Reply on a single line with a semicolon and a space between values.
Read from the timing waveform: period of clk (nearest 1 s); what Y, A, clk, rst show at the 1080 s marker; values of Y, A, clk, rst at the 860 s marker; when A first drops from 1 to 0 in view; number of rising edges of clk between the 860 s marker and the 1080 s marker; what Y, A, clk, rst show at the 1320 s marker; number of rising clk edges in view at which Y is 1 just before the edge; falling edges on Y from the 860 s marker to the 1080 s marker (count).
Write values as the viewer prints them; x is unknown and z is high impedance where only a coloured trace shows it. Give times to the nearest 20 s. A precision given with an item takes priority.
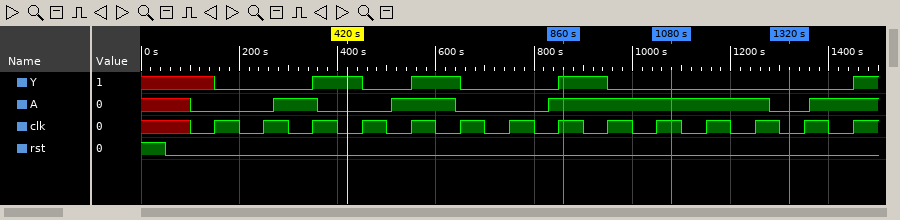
100 s; Y=0, A=1, clk=1, rst=0; Y=1, A=1, clk=1, rst=0; 360 s; 2; Y=0, A=0, clk=0, rst=0; 3; 1
